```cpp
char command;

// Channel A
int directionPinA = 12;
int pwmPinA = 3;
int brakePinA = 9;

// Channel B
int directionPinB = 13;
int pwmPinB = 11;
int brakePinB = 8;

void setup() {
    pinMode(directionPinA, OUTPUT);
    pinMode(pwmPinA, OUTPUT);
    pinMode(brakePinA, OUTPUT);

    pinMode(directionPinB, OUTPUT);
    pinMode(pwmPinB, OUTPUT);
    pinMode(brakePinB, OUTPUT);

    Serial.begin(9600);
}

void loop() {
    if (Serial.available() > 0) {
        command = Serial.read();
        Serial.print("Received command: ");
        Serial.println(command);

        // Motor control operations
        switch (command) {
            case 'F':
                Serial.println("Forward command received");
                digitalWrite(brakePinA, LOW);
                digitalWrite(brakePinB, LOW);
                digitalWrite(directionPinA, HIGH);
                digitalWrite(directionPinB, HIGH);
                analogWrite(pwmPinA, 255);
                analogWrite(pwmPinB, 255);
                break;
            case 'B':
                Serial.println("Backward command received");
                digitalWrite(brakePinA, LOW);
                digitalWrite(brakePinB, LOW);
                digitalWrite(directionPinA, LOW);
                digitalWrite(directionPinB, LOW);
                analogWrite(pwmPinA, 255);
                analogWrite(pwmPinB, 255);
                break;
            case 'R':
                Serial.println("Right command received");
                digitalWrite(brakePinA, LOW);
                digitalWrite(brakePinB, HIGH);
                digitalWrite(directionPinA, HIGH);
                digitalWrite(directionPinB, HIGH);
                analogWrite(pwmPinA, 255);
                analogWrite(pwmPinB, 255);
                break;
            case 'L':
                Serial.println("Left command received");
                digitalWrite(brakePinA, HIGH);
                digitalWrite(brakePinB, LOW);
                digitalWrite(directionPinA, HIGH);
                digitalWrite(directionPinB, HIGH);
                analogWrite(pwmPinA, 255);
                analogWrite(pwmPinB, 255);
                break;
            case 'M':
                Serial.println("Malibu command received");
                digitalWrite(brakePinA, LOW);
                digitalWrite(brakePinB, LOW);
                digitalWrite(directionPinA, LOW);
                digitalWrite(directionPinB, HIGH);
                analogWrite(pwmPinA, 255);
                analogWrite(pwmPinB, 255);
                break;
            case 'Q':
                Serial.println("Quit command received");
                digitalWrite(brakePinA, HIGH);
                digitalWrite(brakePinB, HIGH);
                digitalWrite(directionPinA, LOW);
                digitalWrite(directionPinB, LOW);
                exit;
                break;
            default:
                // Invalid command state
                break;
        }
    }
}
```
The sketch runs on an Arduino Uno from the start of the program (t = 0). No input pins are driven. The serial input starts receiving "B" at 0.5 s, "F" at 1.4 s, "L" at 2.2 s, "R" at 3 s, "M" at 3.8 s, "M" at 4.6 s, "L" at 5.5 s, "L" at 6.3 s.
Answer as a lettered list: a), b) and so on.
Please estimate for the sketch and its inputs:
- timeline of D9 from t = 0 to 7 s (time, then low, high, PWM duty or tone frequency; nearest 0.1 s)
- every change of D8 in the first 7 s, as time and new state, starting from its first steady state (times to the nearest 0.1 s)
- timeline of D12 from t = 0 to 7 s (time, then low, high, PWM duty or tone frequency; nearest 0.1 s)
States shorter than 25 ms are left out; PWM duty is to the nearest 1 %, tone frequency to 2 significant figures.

a) 0 s low; 2.2 s high; 3 s low; 5.5 s high
b) 0 s low; 3 s high; 3.8 s low
c) 0 s low; 1.4 s high; 3.8 s low; 5.5 s high
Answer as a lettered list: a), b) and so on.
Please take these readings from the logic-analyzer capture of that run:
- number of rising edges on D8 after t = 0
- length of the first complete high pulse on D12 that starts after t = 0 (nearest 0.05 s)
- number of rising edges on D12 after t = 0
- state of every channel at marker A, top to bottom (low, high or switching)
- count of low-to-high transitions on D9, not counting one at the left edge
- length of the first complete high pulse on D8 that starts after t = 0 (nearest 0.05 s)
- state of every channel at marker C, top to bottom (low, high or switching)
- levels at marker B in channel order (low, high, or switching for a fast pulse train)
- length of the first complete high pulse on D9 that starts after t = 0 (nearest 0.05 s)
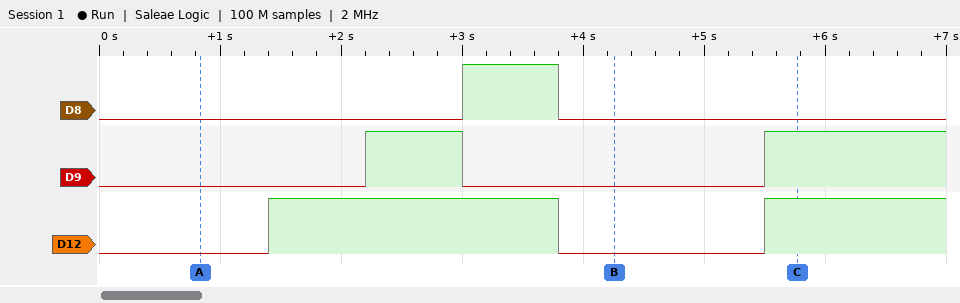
a) 1
b) 2.40 s
c) 2
d) D8 low, D9 low, D12 low
e) 2
f) 0.80 s
g) D8 low, D9 high, D12 high
h) D8 low, D9 low, D12 low
i) 0.80 s
